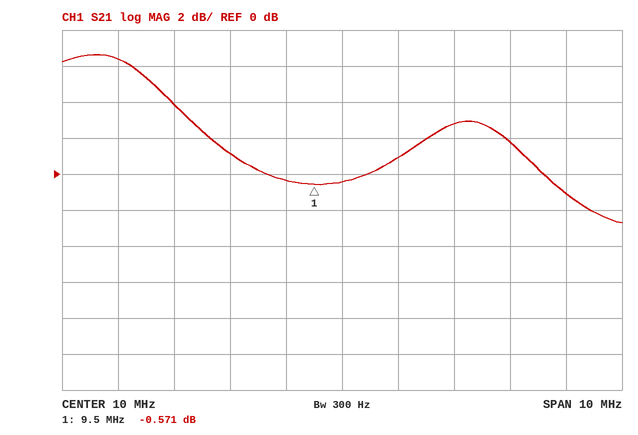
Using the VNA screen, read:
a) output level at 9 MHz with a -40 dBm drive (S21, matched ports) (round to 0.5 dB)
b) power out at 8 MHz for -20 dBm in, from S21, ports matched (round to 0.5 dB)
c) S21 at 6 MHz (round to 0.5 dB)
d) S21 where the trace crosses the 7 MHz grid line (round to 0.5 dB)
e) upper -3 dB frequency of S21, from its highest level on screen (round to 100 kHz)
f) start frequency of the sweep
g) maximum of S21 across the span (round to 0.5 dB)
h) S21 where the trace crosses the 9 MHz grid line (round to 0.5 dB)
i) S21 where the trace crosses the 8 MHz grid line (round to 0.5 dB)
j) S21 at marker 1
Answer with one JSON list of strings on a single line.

["-40.5 dBm", "-19.0 dBm", "6.5 dB", "4.0 dB", "7.1 MHz", "5 MHz", "6.5 dB", "-0.5 dB", "1.0 dB", "-0.571 dB"]
